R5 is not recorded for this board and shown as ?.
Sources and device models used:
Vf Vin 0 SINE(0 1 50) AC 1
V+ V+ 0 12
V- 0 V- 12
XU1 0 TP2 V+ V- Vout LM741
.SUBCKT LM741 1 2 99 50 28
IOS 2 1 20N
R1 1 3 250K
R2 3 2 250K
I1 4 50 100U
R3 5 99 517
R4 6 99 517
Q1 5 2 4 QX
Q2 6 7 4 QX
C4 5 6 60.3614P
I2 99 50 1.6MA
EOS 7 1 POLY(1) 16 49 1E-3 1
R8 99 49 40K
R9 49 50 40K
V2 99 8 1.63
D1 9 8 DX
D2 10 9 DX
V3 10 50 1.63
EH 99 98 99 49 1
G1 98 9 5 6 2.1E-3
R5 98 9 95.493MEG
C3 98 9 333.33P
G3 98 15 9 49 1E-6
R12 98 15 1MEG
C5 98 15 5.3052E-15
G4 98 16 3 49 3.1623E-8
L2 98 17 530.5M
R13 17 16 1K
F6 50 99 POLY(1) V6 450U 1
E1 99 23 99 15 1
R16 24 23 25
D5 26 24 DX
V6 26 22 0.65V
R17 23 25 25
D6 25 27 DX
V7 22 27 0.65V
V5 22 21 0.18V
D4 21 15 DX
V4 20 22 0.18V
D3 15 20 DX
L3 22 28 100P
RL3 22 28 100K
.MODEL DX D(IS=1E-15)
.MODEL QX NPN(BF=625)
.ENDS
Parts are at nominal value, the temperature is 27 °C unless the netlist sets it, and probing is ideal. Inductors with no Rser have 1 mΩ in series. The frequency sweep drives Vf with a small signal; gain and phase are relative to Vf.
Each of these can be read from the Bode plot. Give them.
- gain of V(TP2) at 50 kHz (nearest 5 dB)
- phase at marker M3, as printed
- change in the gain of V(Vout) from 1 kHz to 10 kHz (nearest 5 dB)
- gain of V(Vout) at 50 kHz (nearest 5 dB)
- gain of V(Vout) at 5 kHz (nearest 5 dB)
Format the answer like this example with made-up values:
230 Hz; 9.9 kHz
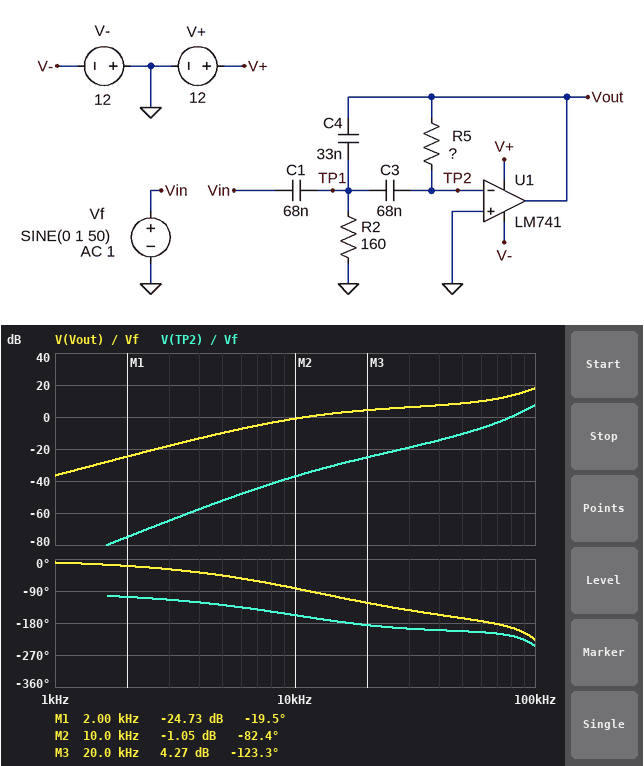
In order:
-10 dB; -123.3 deg; 35 dB; 10 dB; -10 dB
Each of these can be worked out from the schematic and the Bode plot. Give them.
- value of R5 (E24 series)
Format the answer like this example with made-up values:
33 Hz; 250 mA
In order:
510 Ω
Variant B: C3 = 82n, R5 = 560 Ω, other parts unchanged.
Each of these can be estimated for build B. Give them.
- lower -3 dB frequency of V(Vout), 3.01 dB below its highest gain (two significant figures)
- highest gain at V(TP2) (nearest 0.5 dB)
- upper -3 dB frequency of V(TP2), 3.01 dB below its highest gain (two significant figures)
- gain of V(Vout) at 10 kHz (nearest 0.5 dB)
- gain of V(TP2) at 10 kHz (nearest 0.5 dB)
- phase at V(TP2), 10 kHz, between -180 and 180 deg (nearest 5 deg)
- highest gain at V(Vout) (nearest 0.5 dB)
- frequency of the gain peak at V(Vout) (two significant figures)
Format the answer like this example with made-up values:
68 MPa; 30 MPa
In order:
91 kHz; 9.5 dB; 150 kHz; 1.0 dB; -35.5 dB; -165 deg; 18.5 dB; 110 kHz
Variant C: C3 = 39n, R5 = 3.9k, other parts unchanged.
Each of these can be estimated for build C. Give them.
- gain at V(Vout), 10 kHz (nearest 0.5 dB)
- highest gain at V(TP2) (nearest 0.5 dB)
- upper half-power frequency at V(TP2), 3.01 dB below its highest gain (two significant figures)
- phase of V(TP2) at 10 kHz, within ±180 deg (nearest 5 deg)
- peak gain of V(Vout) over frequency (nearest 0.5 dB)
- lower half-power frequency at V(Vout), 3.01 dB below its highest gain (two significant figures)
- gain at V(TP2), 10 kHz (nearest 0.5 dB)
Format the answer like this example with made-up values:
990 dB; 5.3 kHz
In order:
8.0 dB; 8.5 dB; 160 kHz; 140 deg; 17.5 dB; 90 kHz; -31.0 dB
